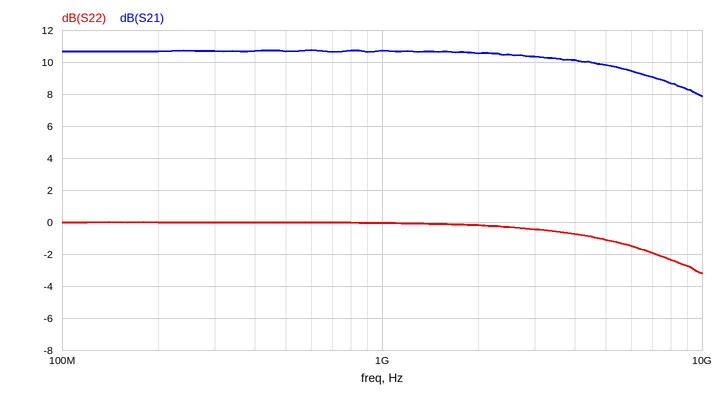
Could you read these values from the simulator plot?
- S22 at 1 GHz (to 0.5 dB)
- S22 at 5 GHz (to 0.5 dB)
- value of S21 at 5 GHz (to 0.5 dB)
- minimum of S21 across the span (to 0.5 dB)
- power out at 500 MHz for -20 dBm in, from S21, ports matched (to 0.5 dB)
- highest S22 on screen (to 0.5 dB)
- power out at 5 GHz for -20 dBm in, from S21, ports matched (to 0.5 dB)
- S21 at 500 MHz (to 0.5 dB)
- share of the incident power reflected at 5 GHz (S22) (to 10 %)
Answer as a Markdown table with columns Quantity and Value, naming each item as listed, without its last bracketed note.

| Quantity | Value |
|---|---|
| S22 at 1 GHz | 0.0 dB |
| S22 at 5 GHz | -1.0 dB |
| value of S21 at 5 GHz | 10.0 dB |
| minimum of S21 across the span | 8.0 dB |
| power out at 500 MHz for -20 dBm in, from S21, ports matched | -9.5 dBm |
| highest S22 on screen | 0.0 dB |
| power out at 5 GHz for -20 dBm in, from S21, ports matched | -10.0 dBm |
| S21 at 500 MHz | 10.5 dB |
| share of the incident power reflected at 5 GHz (S22) | 80 % |
